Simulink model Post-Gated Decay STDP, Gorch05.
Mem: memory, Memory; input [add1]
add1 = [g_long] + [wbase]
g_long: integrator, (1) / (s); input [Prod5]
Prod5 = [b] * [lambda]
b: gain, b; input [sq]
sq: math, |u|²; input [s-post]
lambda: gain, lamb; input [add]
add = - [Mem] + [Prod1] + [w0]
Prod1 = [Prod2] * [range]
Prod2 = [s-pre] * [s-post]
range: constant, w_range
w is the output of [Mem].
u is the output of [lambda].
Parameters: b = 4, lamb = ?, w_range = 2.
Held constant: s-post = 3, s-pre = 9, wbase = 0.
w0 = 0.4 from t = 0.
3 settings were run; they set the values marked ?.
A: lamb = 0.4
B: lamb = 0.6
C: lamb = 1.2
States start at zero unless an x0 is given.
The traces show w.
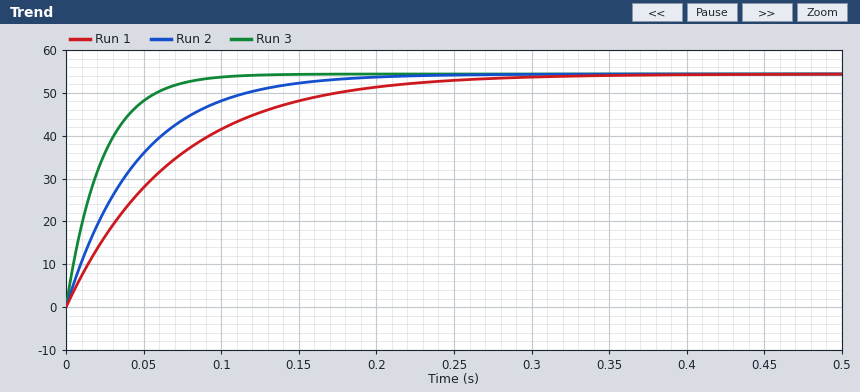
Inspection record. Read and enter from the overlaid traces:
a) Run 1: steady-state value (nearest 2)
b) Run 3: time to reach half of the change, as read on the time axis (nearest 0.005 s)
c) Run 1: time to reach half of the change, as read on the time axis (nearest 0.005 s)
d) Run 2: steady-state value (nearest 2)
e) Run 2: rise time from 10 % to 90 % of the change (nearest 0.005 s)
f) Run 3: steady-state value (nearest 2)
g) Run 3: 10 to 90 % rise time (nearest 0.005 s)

54
0.015 s
0.050 s
54
0.100 s
54
0.050 s
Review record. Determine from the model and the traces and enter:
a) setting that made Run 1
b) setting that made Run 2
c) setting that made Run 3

A
B
C
